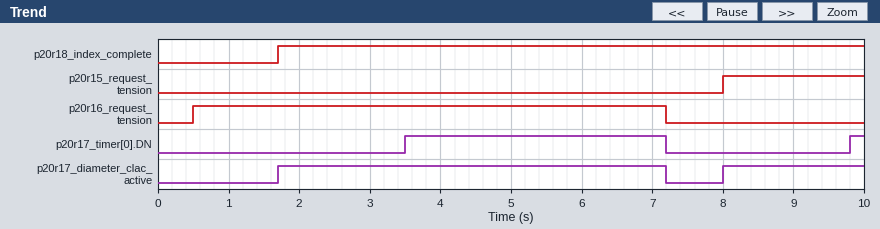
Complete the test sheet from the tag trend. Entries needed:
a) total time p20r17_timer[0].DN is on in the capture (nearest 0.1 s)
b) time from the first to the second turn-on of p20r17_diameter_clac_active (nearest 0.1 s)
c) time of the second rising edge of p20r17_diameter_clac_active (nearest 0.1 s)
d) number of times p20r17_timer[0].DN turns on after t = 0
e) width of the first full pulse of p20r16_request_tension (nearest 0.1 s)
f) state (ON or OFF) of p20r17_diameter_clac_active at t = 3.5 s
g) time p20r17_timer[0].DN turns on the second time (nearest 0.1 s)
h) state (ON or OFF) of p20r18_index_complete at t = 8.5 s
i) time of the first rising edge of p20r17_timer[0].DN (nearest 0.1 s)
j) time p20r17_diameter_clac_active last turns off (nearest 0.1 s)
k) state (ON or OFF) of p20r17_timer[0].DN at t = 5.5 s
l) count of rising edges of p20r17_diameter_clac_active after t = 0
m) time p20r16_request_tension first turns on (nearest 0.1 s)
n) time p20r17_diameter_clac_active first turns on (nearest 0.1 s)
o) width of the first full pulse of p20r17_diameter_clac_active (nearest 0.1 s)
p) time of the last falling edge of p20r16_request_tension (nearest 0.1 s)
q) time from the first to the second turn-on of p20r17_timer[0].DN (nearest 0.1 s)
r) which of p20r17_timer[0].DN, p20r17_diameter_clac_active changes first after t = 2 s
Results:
3.9 s
6.3 s
8.0 s
2
6.7 s
ON
9.8 s
ON
3.5 s
7.2 s
ON
2
0.5 s
1.7 s
5.5 s
7.2 s
6.3 s
p20r17_timer[0].DN
